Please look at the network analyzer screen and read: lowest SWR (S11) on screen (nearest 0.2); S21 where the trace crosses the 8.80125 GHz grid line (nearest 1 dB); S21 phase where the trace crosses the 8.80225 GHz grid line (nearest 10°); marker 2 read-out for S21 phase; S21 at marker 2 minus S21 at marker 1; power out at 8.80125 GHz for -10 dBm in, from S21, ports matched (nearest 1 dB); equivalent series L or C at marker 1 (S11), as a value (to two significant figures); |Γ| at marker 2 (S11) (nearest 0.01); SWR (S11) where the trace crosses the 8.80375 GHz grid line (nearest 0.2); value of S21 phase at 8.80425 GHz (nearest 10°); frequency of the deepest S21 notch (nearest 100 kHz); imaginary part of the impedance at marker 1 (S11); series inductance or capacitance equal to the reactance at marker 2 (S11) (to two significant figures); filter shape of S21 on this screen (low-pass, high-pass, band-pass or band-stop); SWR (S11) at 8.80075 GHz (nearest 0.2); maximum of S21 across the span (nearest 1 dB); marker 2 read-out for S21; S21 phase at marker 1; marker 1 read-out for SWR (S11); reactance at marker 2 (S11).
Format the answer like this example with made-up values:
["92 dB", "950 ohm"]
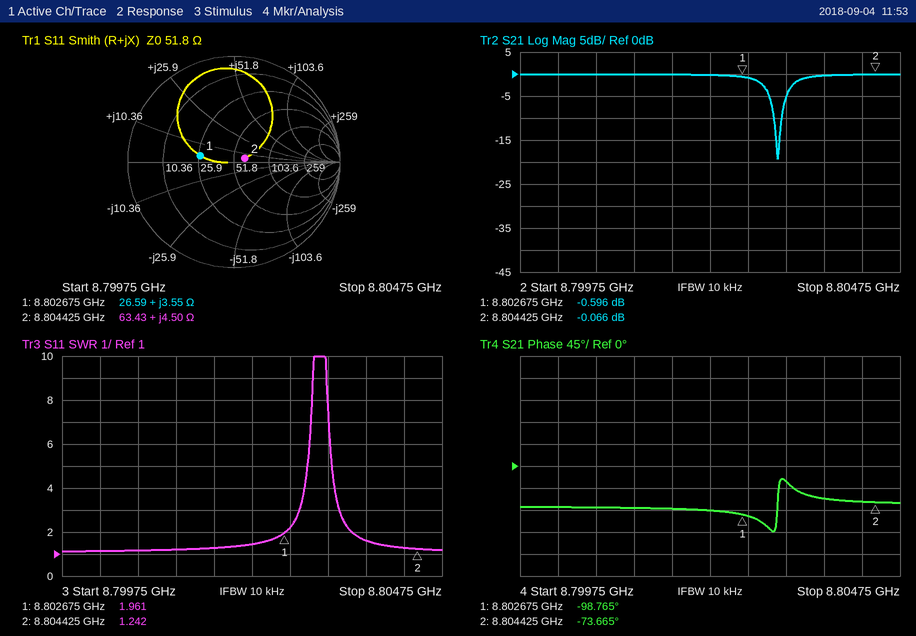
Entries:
["1.2", "0 dB", "-90°", "-73.665°", "0.530 dB", "-10 dBm", "64 pH", "0.11", "1.6", "-70°", "8.8031 GHz", "+3.55 Ω", "81 pH", "band-stop", "1.2", "0 dB", "-0.066 dB", "-98.765°", "1.961", "+4.50 Ω"]
